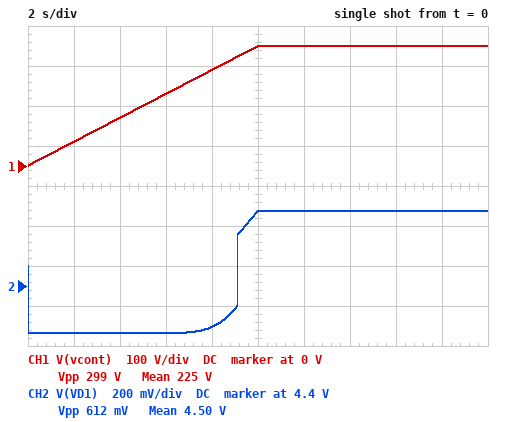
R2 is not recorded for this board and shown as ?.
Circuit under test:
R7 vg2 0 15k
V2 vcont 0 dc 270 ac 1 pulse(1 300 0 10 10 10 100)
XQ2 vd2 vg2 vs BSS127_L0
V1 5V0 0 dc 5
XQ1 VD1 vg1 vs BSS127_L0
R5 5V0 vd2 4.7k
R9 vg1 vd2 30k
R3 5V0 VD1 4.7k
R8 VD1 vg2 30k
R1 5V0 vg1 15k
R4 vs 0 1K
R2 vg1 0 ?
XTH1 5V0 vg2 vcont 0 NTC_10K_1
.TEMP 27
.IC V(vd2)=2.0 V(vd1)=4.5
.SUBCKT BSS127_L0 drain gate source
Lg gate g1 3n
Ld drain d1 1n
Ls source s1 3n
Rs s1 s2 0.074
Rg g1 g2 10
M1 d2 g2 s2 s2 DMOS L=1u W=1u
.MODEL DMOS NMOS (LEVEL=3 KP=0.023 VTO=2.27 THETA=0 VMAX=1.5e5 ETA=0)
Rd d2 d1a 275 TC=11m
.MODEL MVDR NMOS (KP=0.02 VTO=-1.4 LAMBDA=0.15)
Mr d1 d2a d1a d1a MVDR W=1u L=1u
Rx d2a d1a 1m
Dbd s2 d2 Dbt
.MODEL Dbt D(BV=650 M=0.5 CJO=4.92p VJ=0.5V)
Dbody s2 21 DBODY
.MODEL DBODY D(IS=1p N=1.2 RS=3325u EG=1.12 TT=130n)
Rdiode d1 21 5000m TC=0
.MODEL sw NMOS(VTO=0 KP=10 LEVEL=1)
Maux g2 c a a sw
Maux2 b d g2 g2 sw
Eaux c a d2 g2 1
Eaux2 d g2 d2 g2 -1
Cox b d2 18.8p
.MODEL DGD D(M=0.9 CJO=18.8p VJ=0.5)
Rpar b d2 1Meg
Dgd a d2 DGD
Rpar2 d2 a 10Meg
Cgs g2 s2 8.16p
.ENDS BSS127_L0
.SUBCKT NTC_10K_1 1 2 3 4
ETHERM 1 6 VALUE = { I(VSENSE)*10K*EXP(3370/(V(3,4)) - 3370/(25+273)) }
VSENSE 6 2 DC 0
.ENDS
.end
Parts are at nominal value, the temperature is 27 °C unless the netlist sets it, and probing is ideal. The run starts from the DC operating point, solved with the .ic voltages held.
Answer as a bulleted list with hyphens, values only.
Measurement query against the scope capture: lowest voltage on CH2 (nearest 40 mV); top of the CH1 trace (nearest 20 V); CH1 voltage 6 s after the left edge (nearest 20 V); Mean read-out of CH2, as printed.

- 4.16 V
- 300 V
- 180 V
- 4.50 V
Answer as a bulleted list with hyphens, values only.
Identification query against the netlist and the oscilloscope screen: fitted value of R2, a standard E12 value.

- 10 kΩ
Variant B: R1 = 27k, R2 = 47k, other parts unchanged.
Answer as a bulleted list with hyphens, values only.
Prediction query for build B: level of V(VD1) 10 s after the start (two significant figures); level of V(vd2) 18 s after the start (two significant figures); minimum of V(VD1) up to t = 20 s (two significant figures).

- 1.2 V
- 4.8 V
- 1.1 V
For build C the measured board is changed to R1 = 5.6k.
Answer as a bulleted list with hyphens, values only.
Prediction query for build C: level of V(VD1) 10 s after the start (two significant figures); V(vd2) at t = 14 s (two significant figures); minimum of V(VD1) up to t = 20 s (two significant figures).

- 1.4 V
- 4.8 V
- 1.2 V
